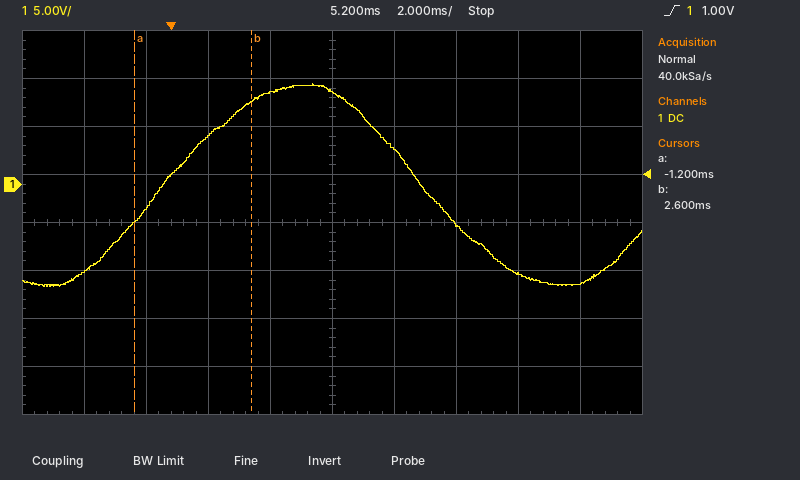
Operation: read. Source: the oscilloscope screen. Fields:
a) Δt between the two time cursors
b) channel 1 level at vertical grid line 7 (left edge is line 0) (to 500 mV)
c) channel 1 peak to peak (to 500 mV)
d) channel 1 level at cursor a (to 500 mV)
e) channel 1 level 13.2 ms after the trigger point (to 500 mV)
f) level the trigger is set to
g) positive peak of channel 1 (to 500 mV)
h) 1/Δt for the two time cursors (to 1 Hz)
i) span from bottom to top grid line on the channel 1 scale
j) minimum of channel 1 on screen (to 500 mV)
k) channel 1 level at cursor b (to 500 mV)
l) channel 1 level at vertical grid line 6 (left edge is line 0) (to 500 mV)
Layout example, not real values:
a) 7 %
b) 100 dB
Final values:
a) 3.8 ms
b) -4.0 V
c) 21.0 V
d) -4.0 V
e) -10.5 V
f) 1.00 V
g) 10.5 V
h) 263 Hz
i) 40 V
j) -10.5 V
k) 8.5 V
l) 3.5 V
